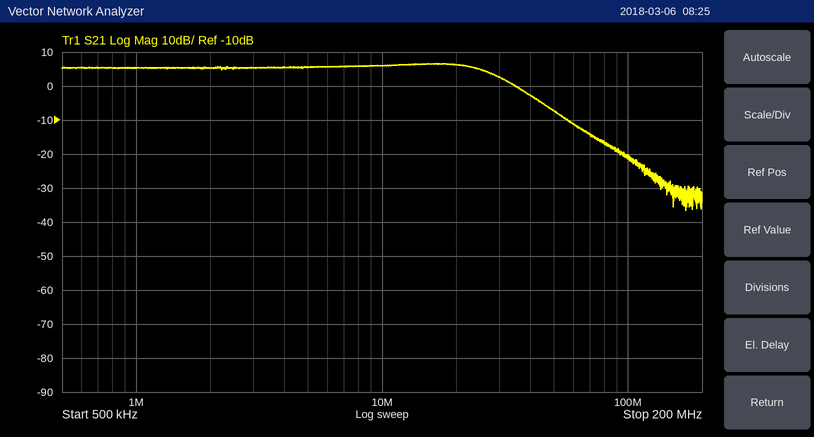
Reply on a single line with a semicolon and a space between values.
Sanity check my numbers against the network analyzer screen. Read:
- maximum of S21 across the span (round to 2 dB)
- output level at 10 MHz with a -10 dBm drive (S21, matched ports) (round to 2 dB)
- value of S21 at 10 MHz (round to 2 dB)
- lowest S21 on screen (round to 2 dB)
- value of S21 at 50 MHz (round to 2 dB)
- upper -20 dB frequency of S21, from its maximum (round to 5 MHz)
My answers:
6 dB; -4 dBm; 6 dB; -36 dB; -8 dB; 65 MHz
